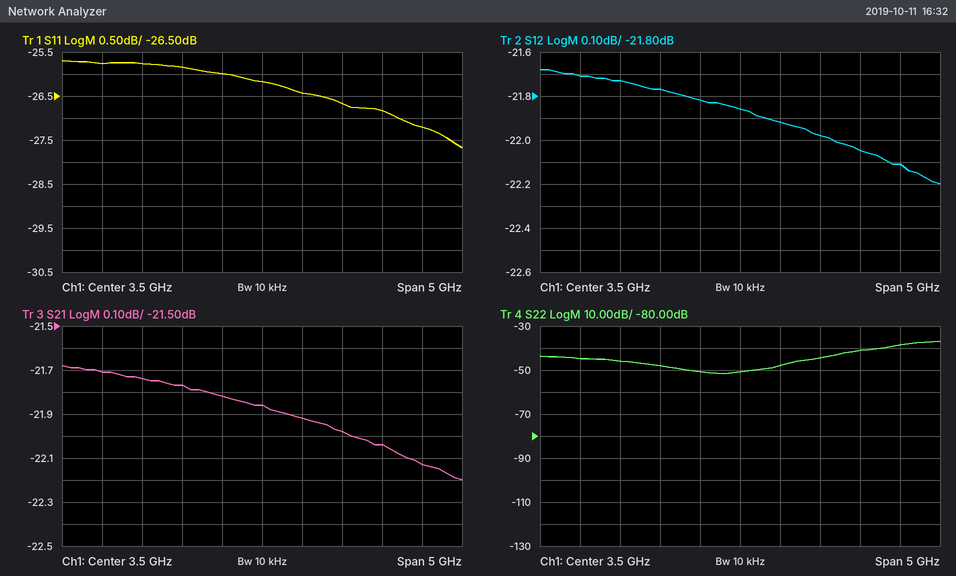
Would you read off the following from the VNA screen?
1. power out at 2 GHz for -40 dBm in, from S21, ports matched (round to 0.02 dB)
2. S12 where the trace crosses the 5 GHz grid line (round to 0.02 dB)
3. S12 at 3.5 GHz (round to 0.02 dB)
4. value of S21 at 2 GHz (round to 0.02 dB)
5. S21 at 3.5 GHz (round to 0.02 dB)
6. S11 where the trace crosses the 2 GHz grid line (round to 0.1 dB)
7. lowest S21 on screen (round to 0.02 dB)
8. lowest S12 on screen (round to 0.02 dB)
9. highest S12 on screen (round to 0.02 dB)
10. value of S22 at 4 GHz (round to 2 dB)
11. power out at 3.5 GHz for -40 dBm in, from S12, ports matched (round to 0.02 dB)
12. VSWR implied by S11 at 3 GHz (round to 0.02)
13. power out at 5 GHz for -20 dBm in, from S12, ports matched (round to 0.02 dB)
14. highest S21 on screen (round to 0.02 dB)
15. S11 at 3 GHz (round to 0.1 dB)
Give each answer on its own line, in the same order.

-61.74 dBm
-22.04 dB
-21.86 dB
-21.74 dB
-21.86 dB
-25.8 dB
-22.20 dB
-22.20 dB
-21.68 dB
-48 dB
-61.86 dBm
1.10
-42.04 dBm
-21.68 dB
-26.0 dB
